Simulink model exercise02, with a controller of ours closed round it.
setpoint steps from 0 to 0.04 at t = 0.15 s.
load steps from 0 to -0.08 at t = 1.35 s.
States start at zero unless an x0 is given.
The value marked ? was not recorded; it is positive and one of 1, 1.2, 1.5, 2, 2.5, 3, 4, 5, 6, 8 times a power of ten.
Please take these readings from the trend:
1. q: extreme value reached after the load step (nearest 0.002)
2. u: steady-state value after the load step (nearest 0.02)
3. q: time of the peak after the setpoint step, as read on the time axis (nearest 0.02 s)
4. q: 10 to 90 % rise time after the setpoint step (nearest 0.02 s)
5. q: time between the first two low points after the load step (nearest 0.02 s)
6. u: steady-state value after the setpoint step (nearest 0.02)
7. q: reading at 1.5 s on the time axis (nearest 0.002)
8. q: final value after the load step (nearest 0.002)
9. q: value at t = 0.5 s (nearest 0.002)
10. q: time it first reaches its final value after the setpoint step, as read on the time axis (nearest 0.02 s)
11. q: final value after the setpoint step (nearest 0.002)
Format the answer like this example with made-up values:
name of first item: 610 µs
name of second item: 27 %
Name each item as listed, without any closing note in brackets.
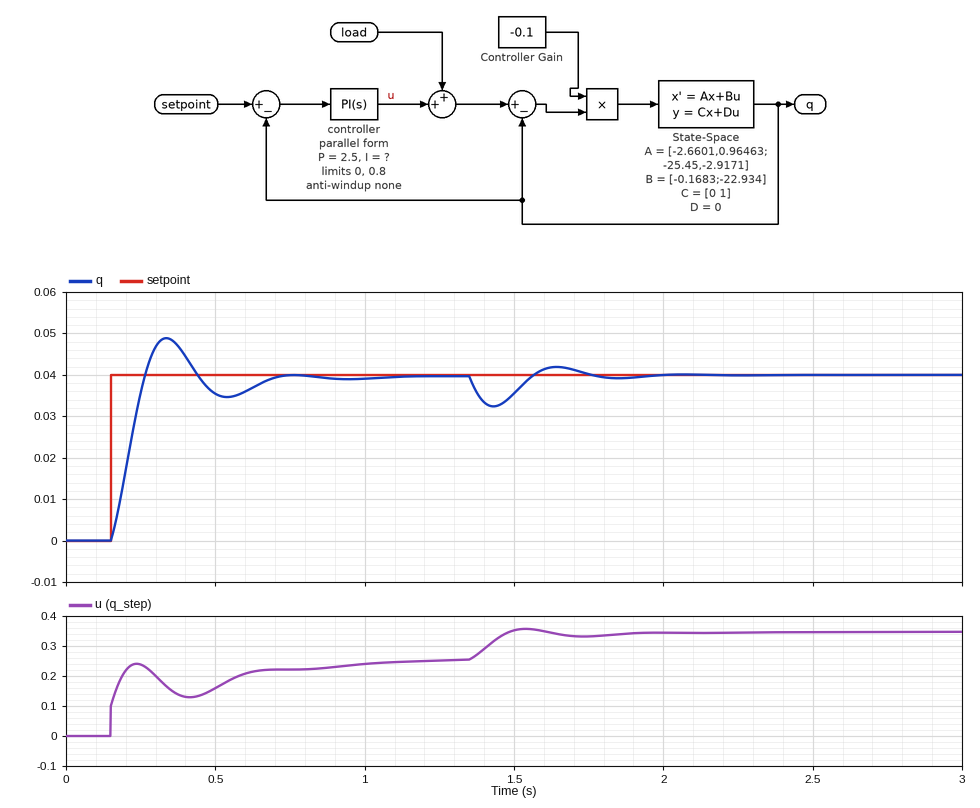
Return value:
q: extreme value reached after the load step: 0.032
u: steady-state value after the load step: 0.34
q: time of the peak after the setpoint step, as read on the time axis: 0.34 s
q: 10 to 90 % rise time after the setpoint step: 0.08 s
q: time between the first two low points after the load step: 0.42 s
u: steady-state value after the setpoint step: 0.26
q: reading at 1.5 s on the time axis: 0.036
q: final value after the load step: 0.040
q: value at t = 0.5 s: 0.036
q: time it first reaches its final value after the setpoint step, as read on the time axis: 0.26 s
q: final value after the setpoint step: 0.040
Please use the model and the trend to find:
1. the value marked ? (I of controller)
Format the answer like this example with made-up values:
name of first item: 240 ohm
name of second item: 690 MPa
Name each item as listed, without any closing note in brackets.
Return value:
the value marked ?: 100
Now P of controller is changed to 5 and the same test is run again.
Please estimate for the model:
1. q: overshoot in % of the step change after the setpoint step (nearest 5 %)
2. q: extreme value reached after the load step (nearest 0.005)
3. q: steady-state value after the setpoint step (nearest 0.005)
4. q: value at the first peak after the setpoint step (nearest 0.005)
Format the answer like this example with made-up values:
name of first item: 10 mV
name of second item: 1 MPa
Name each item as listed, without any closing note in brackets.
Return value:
q: overshoot in % of the step change after the setpoint step: 10 %
q: extreme value reached after the load step: 0.035
q: steady-state value after the setpoint step: 0.040
q: value at the first peak after the setpoint step: 0.045
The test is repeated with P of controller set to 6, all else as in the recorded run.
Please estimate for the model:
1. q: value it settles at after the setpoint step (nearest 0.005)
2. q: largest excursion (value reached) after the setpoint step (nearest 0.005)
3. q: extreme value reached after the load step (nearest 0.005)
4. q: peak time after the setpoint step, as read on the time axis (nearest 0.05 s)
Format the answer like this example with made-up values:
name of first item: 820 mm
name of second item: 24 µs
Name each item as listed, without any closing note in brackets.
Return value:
q: value it settles at after the setpoint step: 0.040
q: largest excursion (value reached) after the setpoint step: 0.045
q: extreme value reached after the load step: 0.035
q: peak time after the setpoint step, as read on the time axis: 0.30 s
